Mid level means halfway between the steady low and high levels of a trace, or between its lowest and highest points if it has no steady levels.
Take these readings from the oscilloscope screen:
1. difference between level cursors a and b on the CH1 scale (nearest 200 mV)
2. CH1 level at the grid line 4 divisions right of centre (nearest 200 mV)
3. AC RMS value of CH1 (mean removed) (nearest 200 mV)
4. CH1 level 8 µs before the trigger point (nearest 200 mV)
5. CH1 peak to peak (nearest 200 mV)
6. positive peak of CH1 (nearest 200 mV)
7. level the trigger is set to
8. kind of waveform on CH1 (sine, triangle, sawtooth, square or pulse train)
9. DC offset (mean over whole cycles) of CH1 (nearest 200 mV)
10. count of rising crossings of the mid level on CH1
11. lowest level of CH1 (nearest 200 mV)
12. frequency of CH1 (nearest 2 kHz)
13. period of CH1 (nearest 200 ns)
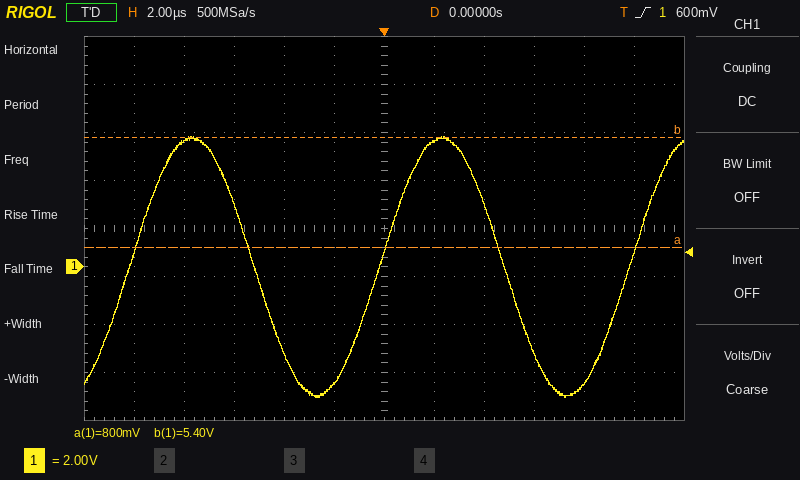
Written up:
4.6 V
-4.8 V
3.8 V
5.2 V
10.8 V
5.4 V
600 mV
sine
0.0 V
3
-5.4 V
100 kHz
10.0 µs
